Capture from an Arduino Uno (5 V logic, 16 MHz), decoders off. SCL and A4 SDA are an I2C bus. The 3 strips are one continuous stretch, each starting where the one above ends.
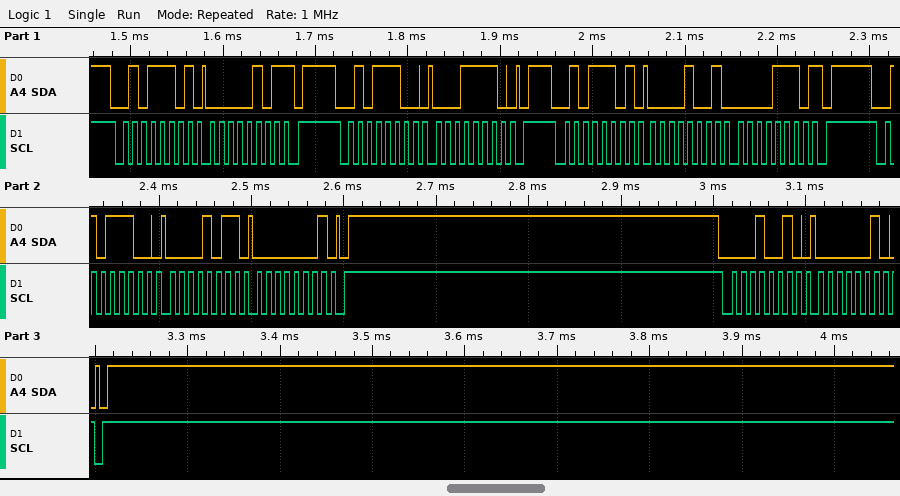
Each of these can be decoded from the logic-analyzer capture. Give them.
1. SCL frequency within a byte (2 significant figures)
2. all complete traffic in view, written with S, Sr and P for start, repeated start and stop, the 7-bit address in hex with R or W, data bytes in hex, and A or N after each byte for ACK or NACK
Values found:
100 kHz
S 2ER A 05 N P S 2EW A 1E A P S 2ER A 09 A 0E N P S 2EW A 0B A 01 A P S 09W A 02 A P
